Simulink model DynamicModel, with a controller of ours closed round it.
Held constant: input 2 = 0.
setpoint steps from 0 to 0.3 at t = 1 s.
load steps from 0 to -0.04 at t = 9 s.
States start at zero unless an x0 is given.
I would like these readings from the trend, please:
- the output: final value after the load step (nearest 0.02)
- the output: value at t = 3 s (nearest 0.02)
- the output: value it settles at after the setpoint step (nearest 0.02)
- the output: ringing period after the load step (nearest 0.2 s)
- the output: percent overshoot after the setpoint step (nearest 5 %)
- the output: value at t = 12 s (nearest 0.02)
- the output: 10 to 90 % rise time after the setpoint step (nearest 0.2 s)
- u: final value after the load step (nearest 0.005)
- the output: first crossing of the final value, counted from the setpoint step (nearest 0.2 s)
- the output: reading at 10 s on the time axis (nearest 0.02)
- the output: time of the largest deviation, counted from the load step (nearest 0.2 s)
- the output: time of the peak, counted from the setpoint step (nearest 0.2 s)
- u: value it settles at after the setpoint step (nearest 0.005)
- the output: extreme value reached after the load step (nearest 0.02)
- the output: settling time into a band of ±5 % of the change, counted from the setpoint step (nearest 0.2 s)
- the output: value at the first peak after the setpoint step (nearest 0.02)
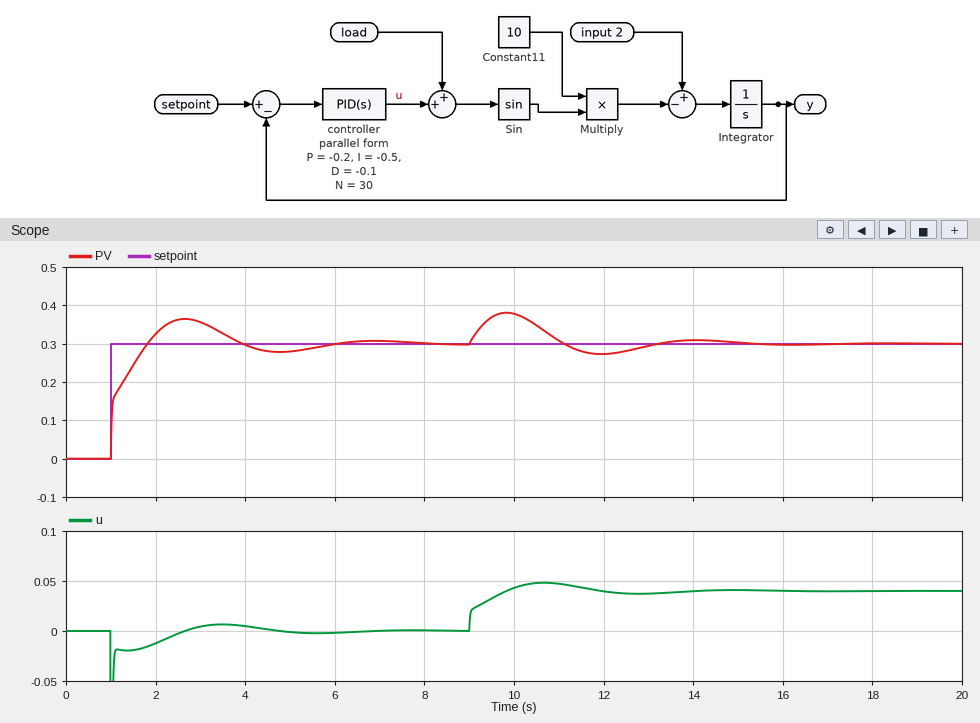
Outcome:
0.30
0.36
0.30
4.2 s
20 %
0.28
0.6 s
0.040
0.8 s
0.38
0.8 s
1.6 s
0.000
0.38
4.4 s
0.36
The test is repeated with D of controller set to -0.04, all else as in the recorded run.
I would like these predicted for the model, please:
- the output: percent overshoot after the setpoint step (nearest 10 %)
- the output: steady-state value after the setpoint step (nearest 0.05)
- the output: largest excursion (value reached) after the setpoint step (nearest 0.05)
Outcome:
30 %
0.30
0.40
